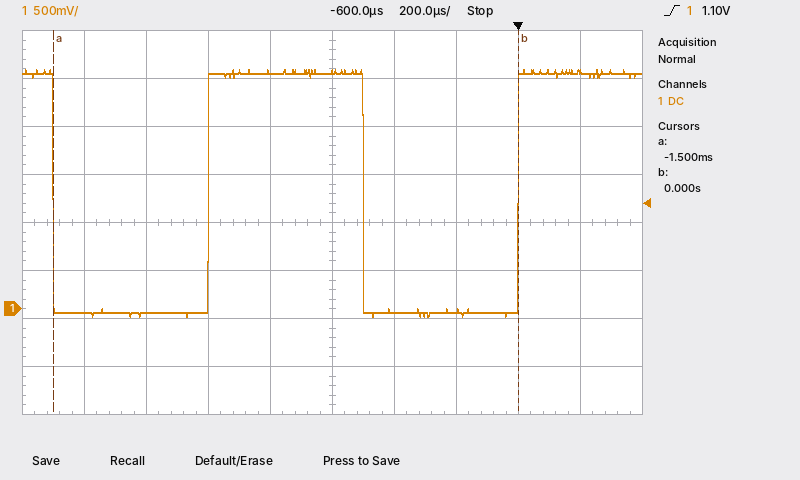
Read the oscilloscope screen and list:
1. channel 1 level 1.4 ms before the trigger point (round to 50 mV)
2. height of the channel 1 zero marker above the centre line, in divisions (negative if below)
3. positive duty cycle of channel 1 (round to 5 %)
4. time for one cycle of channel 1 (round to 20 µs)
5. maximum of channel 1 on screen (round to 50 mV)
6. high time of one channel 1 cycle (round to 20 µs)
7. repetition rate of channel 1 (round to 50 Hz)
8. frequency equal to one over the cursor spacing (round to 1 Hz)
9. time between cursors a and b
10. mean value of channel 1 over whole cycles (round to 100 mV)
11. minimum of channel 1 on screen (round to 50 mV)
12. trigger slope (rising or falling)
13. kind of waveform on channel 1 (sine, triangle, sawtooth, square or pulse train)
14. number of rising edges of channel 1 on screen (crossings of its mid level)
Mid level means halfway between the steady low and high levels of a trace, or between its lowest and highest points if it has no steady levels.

-50 mV
-1.8 div
50 %
1.00 ms
2.50 V
500 µs
1.00 kHz
667 Hz
1.50 ms
1.2 V
-100 mV
rising
square
2
